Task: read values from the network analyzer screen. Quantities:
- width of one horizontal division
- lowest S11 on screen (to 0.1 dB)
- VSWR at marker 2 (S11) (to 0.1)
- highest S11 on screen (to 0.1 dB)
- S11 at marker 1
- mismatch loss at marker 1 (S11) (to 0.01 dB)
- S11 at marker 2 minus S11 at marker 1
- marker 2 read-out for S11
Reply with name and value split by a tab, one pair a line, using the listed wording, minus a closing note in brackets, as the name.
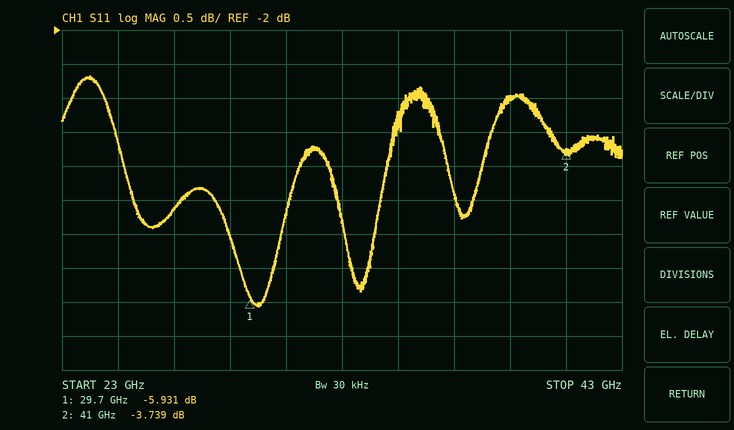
width of one horizontal division	2 GHz
lowest S11 on screen	-6.1 dB
VSWR at marker 2 (S11)	4.7
highest S11 on screen	-2.7 dB
S11 at marker 1	-5.931 dB
mismatch loss at marker 1 (S11)	1.28 dB
S11 at marker 2 minus S11 at marker 1	2.192 dB
marker 2 read-out for S11	-3.739 dB
